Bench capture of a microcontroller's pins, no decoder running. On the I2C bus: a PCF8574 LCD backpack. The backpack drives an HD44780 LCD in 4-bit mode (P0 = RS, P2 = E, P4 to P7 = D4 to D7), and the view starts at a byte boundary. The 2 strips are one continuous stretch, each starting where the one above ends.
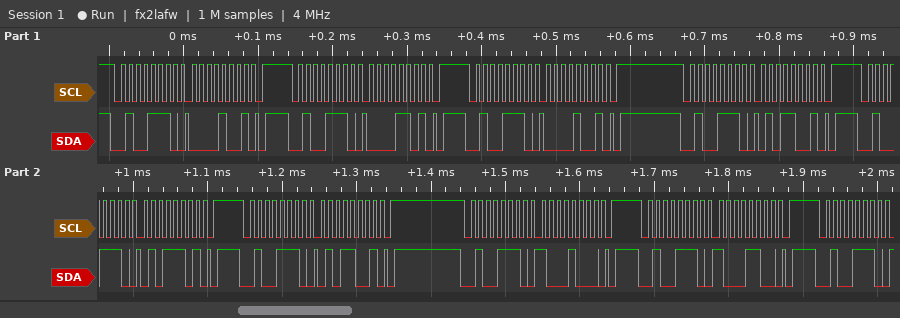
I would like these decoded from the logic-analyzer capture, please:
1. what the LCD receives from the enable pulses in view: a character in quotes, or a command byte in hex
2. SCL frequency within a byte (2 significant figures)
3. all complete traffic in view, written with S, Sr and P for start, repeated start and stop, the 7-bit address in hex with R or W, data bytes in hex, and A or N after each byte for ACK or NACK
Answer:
data 0x05
100 kHz
S 27W A 09 A P S 27W A 0D A P S 27W A 09 A P S 27W A 59 A P S 27W A 5D A P S 27W A 59 A P S 27W A 88 A P S 27W A 8C A P S 27W A
